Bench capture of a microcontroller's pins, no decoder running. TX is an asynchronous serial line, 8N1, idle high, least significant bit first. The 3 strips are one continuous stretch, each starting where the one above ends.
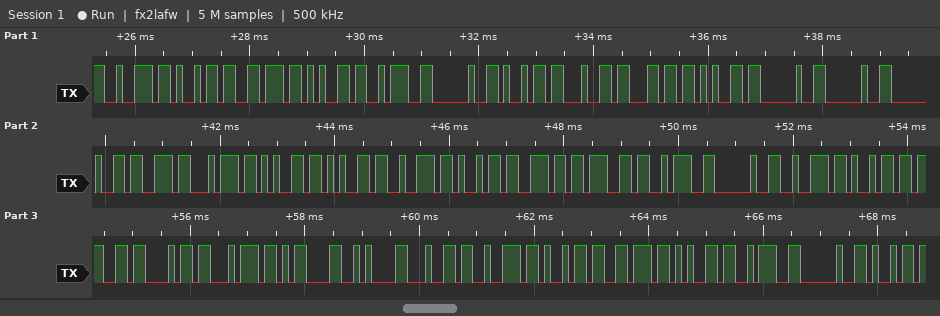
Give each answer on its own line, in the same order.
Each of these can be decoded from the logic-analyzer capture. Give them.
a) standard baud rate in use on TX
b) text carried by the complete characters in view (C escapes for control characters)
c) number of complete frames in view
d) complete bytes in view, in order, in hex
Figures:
9600 baud
"rive: idle   steering: right\r\ndrive: i"
38
72 69 76 65 3A 20 69 64 6C 65 20 20 20 73 74 65 65 72 69 6E 67 3A 20 72 69 67 68 74 0D 0A 64 72 69 76 65 3A 20 69
